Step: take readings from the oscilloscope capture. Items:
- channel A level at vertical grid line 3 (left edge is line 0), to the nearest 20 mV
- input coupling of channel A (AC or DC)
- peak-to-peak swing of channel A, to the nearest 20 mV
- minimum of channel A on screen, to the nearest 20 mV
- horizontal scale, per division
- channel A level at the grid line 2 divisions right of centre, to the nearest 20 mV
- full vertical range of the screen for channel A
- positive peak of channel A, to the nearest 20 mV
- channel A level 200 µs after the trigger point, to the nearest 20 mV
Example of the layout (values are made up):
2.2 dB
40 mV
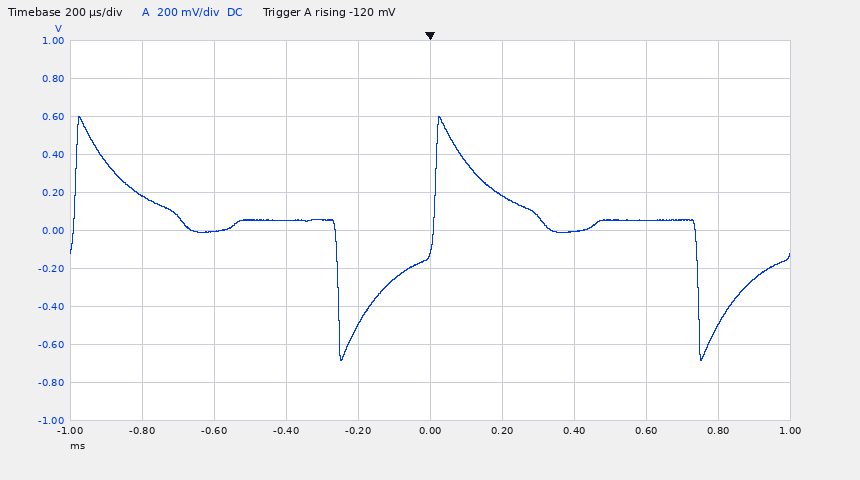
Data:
60 mV
DC
1.28 V
-680 mV
200 µs
0 mV
2 V
600 mV
180 mV
